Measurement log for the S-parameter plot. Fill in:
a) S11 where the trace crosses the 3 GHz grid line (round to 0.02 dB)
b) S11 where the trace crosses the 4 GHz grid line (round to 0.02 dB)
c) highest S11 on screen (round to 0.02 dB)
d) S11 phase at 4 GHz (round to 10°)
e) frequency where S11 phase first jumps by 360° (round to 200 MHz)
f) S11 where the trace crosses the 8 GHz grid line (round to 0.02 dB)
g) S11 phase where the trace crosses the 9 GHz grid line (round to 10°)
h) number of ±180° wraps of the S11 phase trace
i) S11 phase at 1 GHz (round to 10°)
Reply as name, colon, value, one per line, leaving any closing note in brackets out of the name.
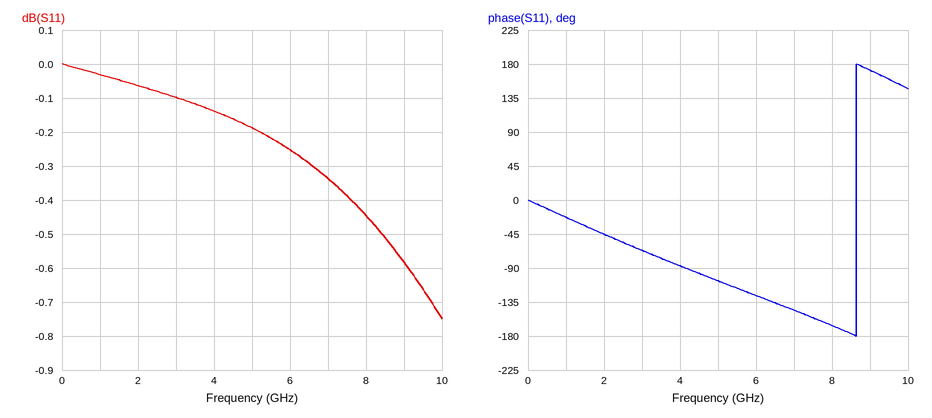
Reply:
S11 where the trace crosses the 3 GHz grid line: -0.10 dB
S11 where the trace crosses the 4 GHz grid line: -0.14 dB
highest S11 on screen: 0.00 dB
S11 phase at 4 GHz: -90°
frequency where S11 phase first jumps by 360°: 8.6 GHz
S11 where the trace crosses the 8 GHz grid line: -0.44 dB
S11 phase where the trace crosses the 9 GHz grid line: 170°
number of ±180° wraps of the S11 phase trace: 1
S11 phase at 1 GHz: -20°
